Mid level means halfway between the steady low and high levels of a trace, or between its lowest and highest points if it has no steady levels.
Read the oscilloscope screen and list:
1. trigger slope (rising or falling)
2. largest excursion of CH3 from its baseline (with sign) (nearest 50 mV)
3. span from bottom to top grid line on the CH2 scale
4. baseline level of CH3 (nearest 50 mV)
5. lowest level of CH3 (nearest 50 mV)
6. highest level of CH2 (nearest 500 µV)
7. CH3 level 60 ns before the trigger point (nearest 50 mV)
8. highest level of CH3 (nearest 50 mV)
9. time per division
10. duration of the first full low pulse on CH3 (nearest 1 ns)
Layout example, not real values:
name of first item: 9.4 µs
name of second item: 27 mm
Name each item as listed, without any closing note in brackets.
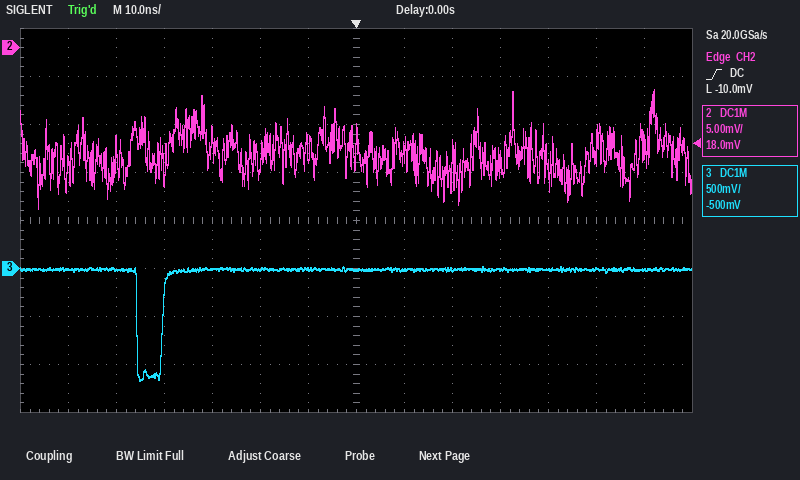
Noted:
trigger slope: rising
largest excursion of CH3 from its baseline (with sign): -1.15 V
span from bottom to top grid line on the CH2 scale: 40 mV
baseline level of CH3: 0 mV
lowest level of CH3: -1.15 V
highest level of CH2: -4.5 mV
CH3 level 60 ns before the trigger point: 0 mV
highest level of CH3: 0 mV
time per division: 10 ns
duration of the first full low pulse on CH3: 5 ns
